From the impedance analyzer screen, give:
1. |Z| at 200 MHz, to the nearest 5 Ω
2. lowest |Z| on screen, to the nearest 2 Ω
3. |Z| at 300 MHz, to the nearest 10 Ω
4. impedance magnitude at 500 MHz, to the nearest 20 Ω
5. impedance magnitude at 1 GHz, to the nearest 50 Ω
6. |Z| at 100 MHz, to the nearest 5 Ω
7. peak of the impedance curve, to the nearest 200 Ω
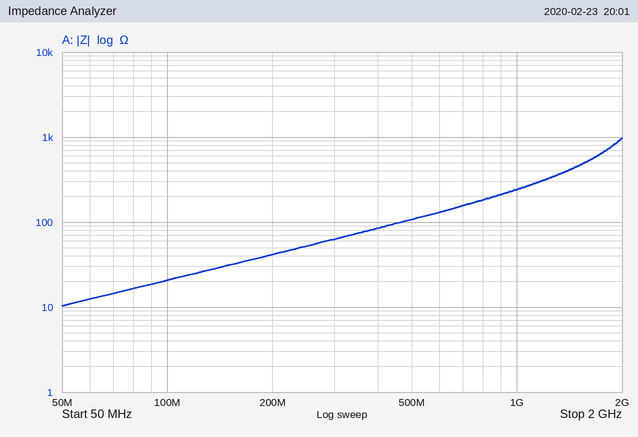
40 Ω
10 Ω
60 Ω
100 Ω
250 Ω
20 Ω
1.0 kΩ
